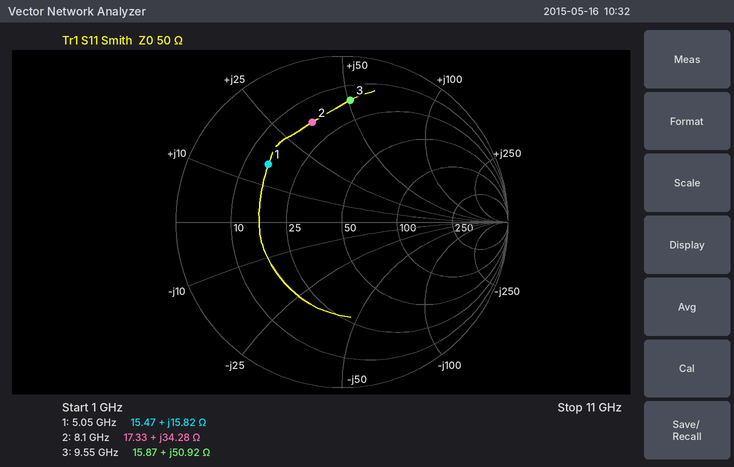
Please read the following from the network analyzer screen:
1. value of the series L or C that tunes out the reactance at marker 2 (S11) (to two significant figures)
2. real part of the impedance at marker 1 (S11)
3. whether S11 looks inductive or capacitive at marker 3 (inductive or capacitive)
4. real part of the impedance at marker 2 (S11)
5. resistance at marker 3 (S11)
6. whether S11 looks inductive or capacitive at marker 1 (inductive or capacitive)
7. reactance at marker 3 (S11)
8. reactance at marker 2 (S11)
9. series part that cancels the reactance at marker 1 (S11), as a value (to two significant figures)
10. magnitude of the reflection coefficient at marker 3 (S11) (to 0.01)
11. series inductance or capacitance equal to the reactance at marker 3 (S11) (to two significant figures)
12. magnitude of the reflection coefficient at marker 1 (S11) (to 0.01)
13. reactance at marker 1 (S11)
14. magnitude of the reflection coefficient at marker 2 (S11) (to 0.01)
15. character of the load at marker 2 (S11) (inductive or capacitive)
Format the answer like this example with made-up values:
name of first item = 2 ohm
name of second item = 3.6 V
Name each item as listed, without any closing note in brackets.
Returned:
value of the series L or C that tunes out the reactance at marker 2 (S11) = 570 fF
real part of the impedance at marker 1 = 15.47 Ω
whether S11 looks inductive or capacitive at marker 3 = inductive
real part of the impedance at marker 2 = 17.33 Ω
resistance at marker 3 = 15.87 Ω
whether S11 looks inductive or capacitive at marker 1 = inductive
reactance at marker 3 = +50.92 Ω
reactance at marker 2 = +34.28 Ω
series part that cancels the reactance at marker 1 (S11), as a value = 2.0 pF
magnitude of the reflection coefficient at marker 3 (S11) = 0.74
series inductance or capacitance equal to the reactance at marker 3 (S11) = 850 pH
magnitude of the reflection coefficient at marker 1 (S11) = 0.56
reactance at marker 1 = +15.82 Ω
magnitude of the reflection coefficient at marker 2 (S11) = 0.63
character of the load at marker 2 (S11) = inductive
